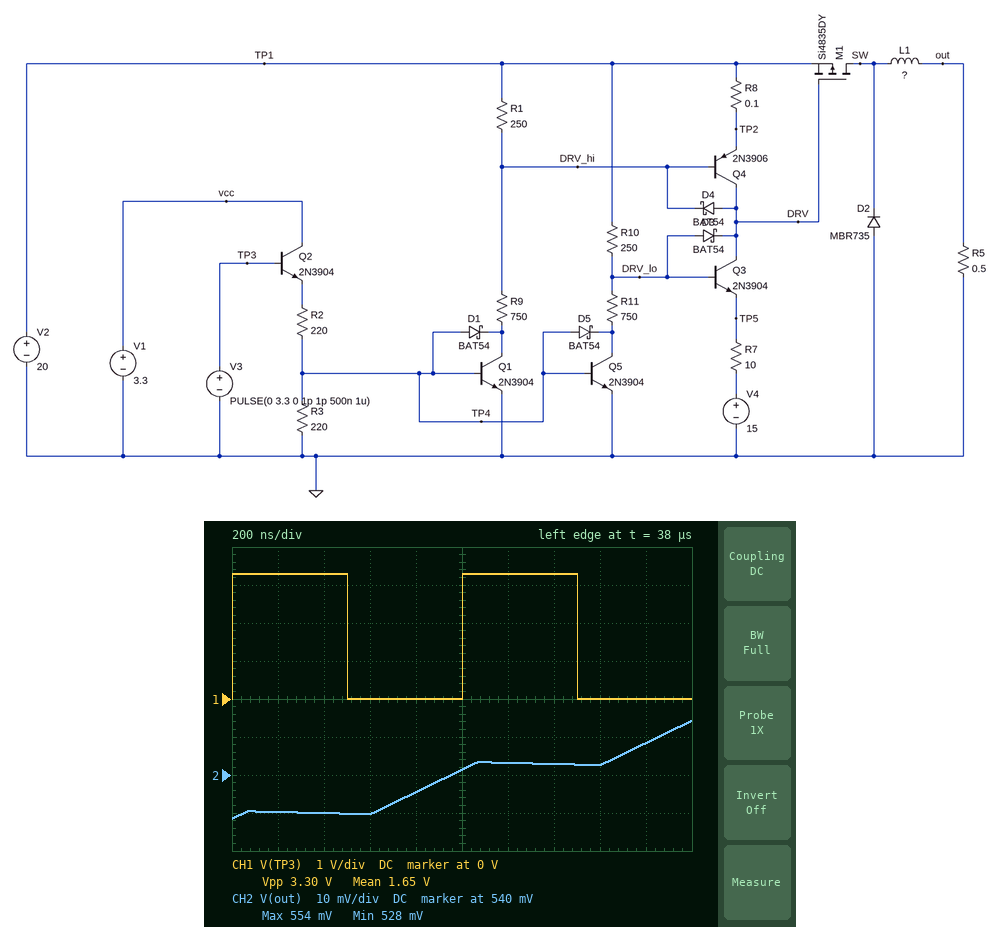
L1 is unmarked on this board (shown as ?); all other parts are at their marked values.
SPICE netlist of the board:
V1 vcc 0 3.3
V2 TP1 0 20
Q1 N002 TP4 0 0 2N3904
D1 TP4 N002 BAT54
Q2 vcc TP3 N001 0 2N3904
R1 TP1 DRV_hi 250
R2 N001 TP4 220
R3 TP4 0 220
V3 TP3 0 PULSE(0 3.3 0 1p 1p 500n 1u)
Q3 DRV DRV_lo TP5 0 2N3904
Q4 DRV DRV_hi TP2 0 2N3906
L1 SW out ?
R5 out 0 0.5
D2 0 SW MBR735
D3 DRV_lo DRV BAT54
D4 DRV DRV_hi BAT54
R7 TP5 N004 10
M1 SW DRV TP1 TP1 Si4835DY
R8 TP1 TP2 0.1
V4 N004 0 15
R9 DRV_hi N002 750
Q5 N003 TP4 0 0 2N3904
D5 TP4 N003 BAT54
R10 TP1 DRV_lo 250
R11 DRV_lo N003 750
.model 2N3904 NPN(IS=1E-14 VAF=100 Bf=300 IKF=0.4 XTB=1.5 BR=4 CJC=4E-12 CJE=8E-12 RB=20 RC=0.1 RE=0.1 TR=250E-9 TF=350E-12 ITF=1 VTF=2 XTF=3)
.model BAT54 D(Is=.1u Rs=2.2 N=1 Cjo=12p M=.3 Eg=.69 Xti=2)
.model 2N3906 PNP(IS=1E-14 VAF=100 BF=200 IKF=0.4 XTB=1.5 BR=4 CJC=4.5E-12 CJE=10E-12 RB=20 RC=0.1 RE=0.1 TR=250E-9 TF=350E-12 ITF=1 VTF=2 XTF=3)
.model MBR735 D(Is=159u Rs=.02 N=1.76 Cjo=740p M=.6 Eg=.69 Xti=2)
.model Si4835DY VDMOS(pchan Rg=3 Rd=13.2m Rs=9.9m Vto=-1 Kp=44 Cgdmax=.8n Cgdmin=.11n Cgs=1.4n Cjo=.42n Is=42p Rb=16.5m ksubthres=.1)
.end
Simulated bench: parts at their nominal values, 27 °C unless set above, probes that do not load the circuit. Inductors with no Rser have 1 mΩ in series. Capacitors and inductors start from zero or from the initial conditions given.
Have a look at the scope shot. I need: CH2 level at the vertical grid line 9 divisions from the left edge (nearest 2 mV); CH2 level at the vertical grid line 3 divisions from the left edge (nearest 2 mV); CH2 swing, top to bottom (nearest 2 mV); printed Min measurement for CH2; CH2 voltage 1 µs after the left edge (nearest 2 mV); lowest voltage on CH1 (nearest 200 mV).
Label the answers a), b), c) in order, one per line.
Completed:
a) 548 mV
b) 530 mV
c) 26 mV
d) 528 mV
e) 542 mV
f) 0 V
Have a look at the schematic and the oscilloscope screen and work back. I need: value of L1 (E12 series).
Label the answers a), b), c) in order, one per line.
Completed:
a) 330 µH
